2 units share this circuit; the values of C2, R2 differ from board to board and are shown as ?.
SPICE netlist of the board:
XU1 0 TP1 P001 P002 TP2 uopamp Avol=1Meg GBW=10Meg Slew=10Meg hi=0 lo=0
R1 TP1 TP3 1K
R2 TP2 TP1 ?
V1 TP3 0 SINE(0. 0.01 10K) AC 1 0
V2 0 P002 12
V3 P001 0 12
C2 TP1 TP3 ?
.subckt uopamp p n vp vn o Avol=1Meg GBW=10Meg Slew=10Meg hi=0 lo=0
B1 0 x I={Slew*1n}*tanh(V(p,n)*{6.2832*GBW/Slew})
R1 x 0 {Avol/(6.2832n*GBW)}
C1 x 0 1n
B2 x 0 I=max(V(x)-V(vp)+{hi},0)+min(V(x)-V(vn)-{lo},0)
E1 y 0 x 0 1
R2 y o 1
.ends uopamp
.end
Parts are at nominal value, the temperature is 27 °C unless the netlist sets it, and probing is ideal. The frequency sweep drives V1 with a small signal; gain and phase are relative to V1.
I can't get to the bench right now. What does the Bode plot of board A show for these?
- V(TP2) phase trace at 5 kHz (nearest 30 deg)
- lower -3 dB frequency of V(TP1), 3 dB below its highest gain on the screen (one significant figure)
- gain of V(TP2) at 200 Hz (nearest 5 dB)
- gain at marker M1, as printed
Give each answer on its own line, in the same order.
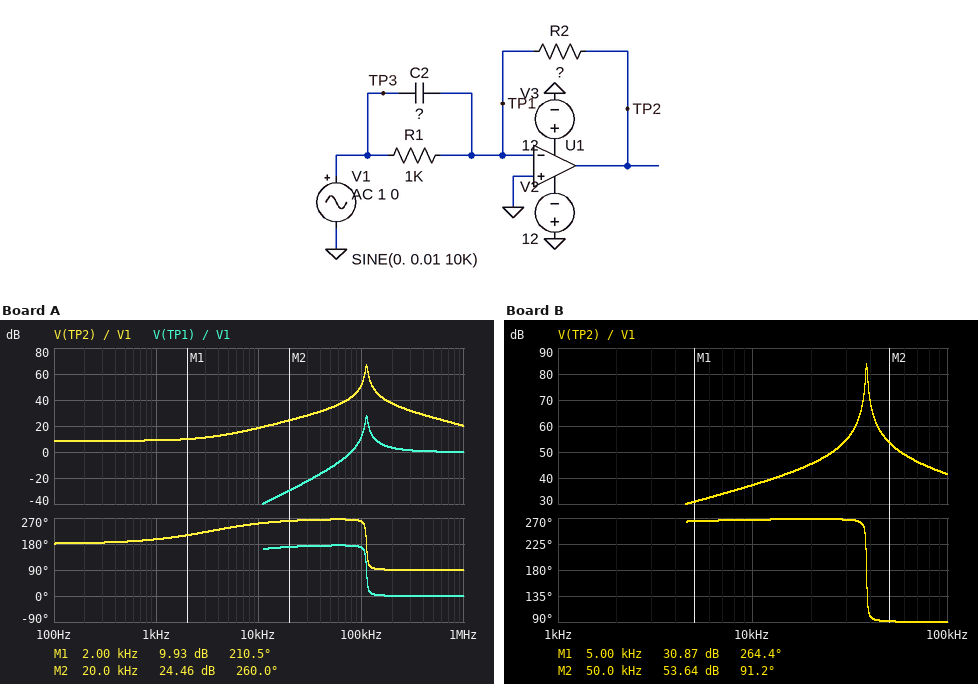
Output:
240 deg
100 kHz
10 dB
9.93 dB
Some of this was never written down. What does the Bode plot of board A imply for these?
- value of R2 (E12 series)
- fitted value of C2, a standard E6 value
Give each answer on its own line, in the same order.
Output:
2.7 kΩ
47 nF
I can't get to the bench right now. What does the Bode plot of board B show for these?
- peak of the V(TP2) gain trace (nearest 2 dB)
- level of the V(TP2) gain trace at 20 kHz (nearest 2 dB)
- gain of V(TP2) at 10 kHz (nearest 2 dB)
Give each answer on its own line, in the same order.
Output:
84 dB
46 dB
38 dB
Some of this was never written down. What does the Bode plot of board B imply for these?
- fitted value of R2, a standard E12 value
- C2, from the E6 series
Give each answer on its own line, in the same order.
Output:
3.3 kΩ
330 nF
